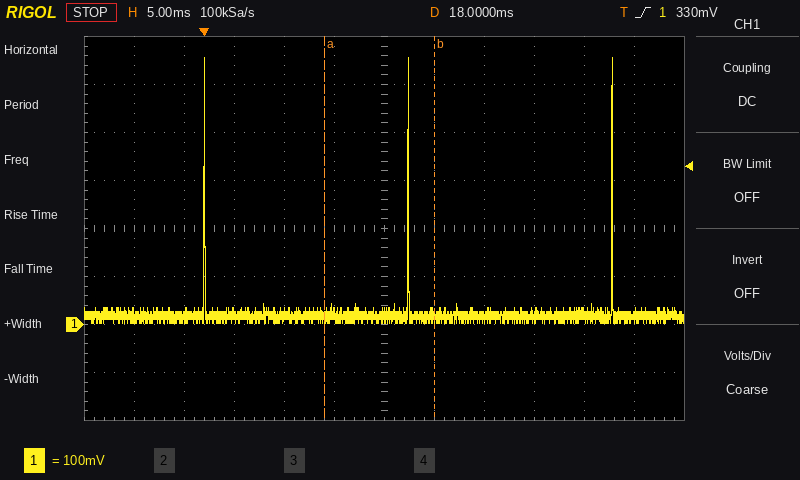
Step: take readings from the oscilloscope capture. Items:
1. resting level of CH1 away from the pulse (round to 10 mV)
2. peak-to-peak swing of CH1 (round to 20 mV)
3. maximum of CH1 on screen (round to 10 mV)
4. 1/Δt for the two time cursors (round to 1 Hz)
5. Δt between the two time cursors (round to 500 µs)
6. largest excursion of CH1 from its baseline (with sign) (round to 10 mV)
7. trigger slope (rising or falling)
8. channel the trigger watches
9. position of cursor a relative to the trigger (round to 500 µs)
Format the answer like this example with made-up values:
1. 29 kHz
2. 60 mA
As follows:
1. 20 mV
2. 560 mV
3. 560 mV
4. 91 Hz
5. 11.0 ms
6. +540 mV
7. rising
8. CH1
9. +12.0 ms
